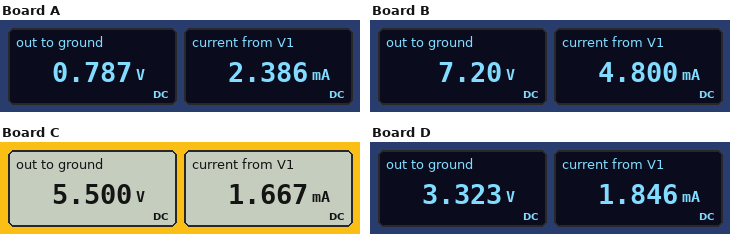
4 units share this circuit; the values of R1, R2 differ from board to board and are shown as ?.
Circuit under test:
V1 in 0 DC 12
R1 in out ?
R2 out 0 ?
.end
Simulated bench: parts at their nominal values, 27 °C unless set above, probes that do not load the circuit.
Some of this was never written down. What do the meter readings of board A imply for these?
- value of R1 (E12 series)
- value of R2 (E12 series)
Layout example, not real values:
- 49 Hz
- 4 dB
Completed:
- 4.7 kΩ
- 330 Ω
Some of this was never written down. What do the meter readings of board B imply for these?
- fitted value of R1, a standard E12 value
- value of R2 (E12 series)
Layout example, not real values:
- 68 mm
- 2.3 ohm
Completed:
- 1 kΩ
- 1.5 kΩ
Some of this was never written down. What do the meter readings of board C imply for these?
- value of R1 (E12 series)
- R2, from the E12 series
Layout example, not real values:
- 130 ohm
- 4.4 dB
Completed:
- 3.9 kΩ
- 3.3 kΩ
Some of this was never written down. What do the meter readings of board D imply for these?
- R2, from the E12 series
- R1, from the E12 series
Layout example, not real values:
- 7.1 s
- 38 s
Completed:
- 1.8 kΩ
- 4.7 kΩ
